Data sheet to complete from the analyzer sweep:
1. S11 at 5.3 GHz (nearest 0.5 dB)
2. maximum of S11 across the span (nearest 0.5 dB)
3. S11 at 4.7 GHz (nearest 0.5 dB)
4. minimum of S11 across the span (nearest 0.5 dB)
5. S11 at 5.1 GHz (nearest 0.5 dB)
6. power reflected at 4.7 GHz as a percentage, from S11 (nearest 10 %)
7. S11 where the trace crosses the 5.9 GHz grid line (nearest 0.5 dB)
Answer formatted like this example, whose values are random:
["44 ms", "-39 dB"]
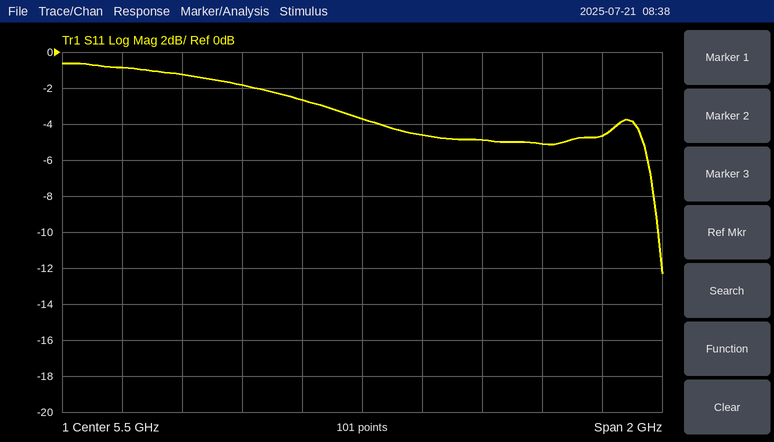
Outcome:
["-2.5 dB", "-0.5 dB", "-1.0 dB", "-12.5 dB", "-2.0 dB", "80 %", "-5.0 dB"]
